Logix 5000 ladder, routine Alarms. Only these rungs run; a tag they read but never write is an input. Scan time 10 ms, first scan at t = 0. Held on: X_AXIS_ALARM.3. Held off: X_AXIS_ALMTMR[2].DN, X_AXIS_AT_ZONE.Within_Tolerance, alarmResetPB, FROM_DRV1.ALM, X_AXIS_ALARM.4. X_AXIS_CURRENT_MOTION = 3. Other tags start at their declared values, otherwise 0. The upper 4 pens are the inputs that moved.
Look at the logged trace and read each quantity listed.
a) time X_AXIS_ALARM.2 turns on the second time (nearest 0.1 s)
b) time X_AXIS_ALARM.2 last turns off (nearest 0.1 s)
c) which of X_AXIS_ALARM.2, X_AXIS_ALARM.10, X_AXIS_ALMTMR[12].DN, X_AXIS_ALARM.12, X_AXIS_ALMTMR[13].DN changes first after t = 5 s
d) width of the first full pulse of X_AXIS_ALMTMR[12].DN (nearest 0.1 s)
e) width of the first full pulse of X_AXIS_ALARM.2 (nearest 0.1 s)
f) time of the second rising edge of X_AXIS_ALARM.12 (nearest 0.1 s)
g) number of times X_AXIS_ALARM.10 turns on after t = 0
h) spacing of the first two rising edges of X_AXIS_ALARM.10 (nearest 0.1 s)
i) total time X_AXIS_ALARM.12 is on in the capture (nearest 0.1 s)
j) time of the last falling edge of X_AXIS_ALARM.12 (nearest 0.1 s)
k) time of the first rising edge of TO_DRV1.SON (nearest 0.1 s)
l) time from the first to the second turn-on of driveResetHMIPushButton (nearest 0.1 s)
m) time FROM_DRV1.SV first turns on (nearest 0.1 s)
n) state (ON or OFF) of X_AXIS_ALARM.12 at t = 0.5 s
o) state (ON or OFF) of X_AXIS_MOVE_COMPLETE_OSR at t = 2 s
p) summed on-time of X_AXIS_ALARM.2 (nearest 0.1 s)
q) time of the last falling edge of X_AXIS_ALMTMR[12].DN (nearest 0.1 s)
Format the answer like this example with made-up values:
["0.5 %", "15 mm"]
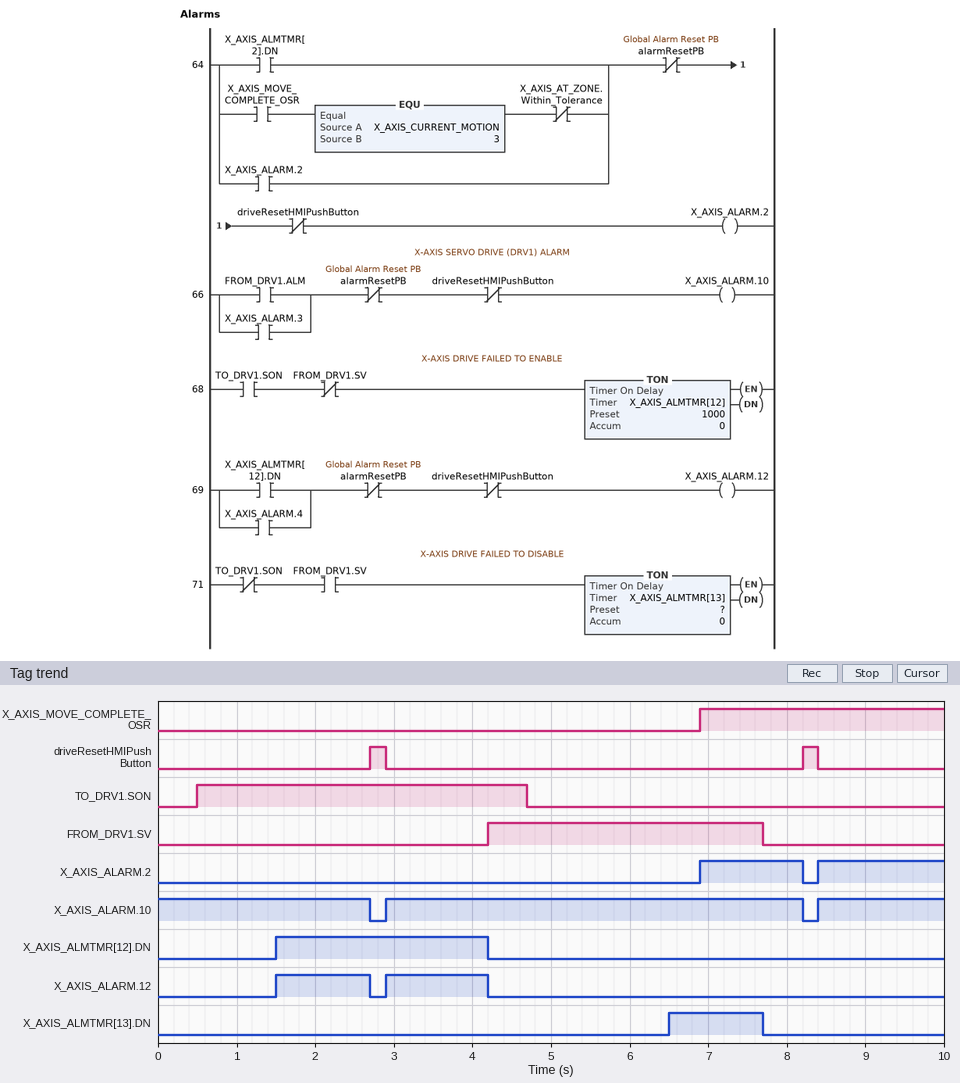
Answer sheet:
["8.4 s", "8.2 s", "X_AXIS_ALMTMR[13].DN", "2.7 s", "1.3 s", "2.9 s", "2", "5.5 s", "2.5 s", "4.2 s", "0.5 s", "5.5 s", "4.2 s", "OFF", "OFF", "2.9 s", "4.2 s"]
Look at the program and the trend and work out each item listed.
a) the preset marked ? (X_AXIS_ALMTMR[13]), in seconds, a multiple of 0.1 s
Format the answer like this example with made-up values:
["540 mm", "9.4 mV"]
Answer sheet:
["1.8 s"]
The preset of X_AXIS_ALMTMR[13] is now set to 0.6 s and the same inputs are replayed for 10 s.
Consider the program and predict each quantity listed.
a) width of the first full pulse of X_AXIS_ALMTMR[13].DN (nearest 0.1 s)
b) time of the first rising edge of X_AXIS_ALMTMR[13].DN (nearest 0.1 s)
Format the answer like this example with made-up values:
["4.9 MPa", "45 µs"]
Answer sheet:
["2.4 s", "5.3 s"]
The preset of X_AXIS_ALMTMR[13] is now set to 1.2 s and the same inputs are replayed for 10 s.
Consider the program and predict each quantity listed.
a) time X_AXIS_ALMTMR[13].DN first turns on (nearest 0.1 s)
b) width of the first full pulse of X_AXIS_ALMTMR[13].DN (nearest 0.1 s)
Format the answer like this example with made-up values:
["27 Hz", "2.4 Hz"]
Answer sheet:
["5.9 s", "1.8 s"]
